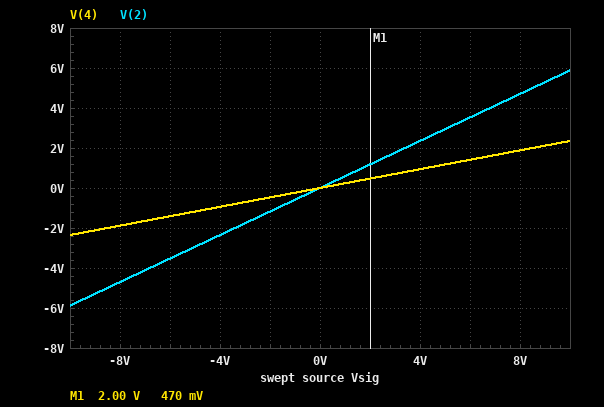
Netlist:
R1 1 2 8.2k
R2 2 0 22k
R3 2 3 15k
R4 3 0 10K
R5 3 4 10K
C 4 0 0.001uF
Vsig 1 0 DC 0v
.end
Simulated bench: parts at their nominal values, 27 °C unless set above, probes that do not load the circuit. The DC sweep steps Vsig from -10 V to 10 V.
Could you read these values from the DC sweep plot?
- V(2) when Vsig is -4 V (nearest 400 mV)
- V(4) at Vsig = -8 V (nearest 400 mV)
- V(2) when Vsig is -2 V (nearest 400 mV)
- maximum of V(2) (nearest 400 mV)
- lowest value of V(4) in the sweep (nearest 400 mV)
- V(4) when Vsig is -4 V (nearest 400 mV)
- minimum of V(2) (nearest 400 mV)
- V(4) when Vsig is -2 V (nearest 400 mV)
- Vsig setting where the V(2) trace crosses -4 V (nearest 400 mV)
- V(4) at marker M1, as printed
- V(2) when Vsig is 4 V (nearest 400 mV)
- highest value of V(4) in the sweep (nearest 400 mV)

-2.4 V
-2.0 V
-1.2 V
6.0 V
-2.4 V
-800 mV
-6.0 V
-400 mV
-6.8 V
470 mV
2.4 V
2.4 V
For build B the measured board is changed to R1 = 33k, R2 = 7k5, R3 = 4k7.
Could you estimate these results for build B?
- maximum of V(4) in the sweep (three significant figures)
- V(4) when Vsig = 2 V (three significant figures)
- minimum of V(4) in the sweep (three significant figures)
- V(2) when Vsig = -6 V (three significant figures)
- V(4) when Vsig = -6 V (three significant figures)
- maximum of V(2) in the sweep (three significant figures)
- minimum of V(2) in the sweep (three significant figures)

890 mV
178 mV
-890 mV
-785 mV
-534 mV
1.31 V
-1.31 V
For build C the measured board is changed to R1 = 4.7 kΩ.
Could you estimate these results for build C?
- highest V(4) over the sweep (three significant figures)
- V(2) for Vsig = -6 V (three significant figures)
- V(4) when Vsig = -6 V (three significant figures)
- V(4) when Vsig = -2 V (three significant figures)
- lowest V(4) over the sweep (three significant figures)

2.85 V
-4.28 V
-1.71 V
-571 mV
-2.85 V
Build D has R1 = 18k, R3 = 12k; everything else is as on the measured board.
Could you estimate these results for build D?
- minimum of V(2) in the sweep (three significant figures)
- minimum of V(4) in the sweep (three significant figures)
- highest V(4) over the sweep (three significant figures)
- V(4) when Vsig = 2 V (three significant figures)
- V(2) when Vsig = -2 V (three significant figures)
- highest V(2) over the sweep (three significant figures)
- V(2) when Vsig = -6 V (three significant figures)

-3.79 V
-1.72 V
1.72 V
345 mV
-759 mV
3.79 V
-2.28 V
